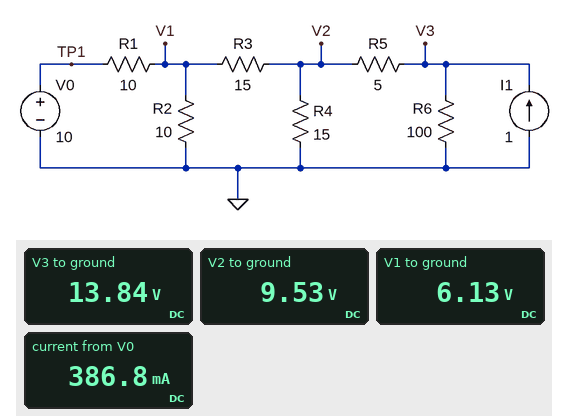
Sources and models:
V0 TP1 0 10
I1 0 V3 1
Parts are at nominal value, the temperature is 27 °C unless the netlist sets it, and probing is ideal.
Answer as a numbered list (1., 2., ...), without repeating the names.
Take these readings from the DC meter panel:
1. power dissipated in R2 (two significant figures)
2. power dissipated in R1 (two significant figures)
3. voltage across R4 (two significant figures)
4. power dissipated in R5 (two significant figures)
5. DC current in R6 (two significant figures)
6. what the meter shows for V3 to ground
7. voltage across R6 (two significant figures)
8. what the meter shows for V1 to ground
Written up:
1. 3.8 W
2. 1.5 W
3. 9.5 V
4. 3.7 W
5. 140 mA
6. 13.84 V
7. 14 V
8. 6.13 V
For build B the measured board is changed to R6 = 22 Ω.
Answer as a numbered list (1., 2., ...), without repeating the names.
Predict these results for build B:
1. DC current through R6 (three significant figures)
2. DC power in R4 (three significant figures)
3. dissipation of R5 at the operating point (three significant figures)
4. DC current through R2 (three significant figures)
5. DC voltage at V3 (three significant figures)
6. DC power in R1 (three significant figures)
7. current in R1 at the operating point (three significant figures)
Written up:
1. 442 mA
2. 3.20 W
3. 1.56 W
4. 548 mA
5. 9.72 V
6. 2.04 W
7. 452 mA
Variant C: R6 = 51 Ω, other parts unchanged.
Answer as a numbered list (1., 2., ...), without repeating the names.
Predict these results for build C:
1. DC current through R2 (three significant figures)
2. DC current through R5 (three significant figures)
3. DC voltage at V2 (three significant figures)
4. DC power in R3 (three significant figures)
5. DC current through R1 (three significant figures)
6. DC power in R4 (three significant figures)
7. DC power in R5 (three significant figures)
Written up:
1. 591 mA
2. 757 mA
3. 8.63 V
4. 494 mW
5. 409 mA
6. 4.96 W
7. 2.86 W
